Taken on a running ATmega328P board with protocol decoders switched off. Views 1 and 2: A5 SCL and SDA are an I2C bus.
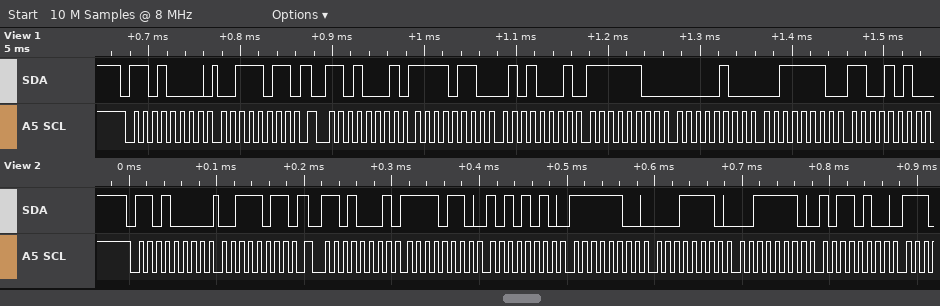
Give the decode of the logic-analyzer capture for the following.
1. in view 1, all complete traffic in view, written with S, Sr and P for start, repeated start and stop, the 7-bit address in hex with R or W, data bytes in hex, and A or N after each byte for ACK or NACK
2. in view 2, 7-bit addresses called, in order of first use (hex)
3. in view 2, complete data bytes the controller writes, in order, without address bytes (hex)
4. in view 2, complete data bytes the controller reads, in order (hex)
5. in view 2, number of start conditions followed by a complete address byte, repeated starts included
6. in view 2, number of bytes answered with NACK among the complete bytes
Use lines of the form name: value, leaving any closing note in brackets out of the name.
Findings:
in view 1, all complete traffic in view, written with S, Sr and P for start, repeated start and stop, the 7-bit address in hex with R or W, data bytes in hex, and A or N after each byte for ACK or NACK: S 68W A 3B A Sr 68R A F6 A 51 A FC A 04 A 3E A CA A
in view 2, 7-bit addresses called, in order of first use: 0x68
in view 2, complete data bytes the controller writes, in order, without address bytes: 3B
in view 2, complete data bytes the controller reads, in order: F6 AA FC 1E 3E B4
in view 2, number of start conditions followed by a complete address byte, repeated starts included: 2
in view 2, number of bytes answered with NACK among the complete bytes: 0
